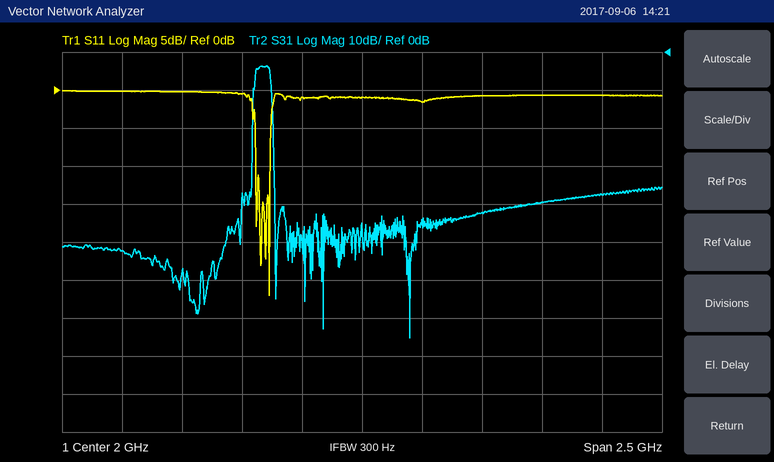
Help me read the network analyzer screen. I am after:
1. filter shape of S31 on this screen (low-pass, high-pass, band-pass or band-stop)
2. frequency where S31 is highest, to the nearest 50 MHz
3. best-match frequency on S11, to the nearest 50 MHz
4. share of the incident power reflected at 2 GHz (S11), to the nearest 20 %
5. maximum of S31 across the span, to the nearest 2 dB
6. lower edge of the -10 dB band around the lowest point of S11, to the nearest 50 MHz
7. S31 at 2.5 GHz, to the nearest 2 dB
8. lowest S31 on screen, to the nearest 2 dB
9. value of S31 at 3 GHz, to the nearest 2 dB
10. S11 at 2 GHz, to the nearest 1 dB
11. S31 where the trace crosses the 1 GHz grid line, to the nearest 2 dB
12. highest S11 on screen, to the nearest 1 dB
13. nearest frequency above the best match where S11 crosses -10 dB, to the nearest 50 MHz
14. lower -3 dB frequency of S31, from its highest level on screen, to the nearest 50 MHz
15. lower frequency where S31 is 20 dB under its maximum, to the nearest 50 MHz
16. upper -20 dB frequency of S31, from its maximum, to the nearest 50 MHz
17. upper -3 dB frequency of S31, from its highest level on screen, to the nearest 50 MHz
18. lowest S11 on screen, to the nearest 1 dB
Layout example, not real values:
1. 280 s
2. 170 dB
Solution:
1. band-pass
2. 1.60 GHz
3. 1.60 GHz
4. 80 %
5. -4 dB
6. 1.55 GHz
7. -42 dB
8. -76 dB
9. -38 dB
10. -1 dB
11. -52 dB
12. 0 dB
13. 1.60 GHz
14. 1.55 GHz
15. 1.55 GHz
16. 1.65 GHz
17. 1.60 GHz
18. -27 dB
